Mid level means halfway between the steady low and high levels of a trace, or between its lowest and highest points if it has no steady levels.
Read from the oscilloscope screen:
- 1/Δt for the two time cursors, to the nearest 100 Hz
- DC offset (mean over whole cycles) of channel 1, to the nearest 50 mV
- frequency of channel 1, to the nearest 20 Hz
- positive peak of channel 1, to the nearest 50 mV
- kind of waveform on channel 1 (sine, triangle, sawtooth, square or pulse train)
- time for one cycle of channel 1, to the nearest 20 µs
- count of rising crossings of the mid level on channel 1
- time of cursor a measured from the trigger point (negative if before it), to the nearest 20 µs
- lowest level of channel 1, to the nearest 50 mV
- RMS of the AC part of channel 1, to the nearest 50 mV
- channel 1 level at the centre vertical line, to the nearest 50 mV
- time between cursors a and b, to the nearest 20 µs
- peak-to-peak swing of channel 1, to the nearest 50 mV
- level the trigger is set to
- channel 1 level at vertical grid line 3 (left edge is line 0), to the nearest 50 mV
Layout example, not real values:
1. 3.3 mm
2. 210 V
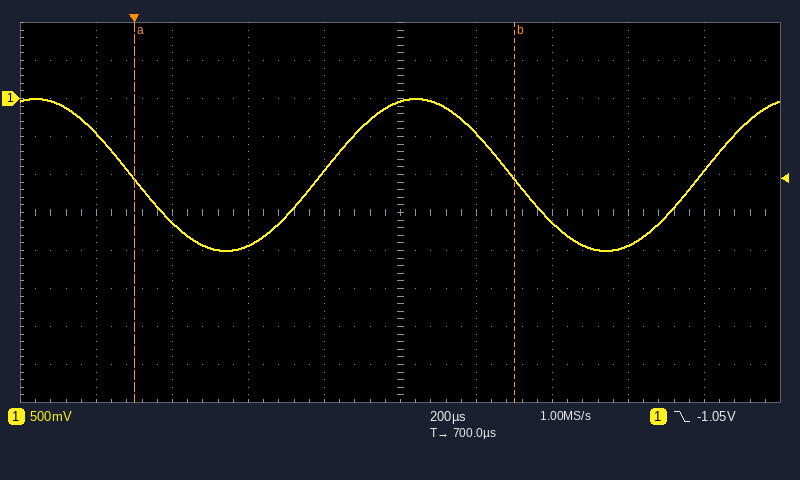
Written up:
1. 1.0 kHz
2. -1.00 V
3. 1.00 kHz
4. 0 mV
5. sine
6. 1.00 ms
7. 2
8. 0 µs
9. -2.00 V
10. 700 mV
11. -50 mV
12. 1.00 ms
13. 2.00 V
14. -1.05 V
15. -1.95 V
